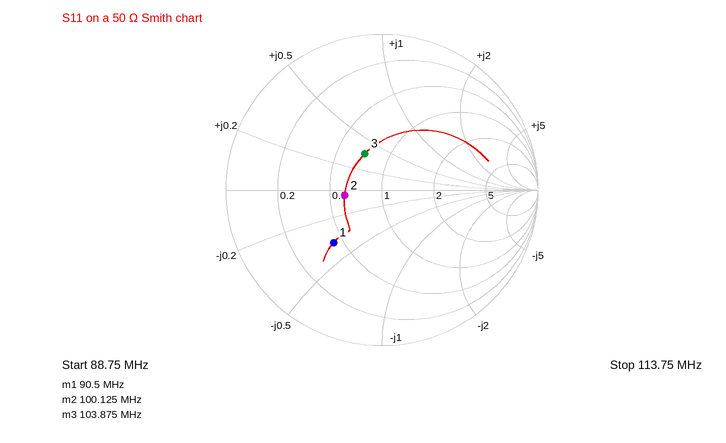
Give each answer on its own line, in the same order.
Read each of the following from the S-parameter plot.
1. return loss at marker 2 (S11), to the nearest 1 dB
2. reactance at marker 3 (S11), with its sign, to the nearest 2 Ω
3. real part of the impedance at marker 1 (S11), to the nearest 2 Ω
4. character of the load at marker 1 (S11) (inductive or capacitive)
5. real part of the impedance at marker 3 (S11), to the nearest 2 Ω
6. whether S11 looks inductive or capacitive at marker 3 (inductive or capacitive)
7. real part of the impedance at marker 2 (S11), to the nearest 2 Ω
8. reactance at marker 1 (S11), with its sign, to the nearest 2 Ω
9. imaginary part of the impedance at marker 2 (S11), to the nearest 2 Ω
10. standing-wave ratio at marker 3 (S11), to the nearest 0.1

12 dB
+18 Ω
22 Ω
capacitive
36 Ω
inductive
30 Ω
-18 Ω
-2 Ω
1.7
